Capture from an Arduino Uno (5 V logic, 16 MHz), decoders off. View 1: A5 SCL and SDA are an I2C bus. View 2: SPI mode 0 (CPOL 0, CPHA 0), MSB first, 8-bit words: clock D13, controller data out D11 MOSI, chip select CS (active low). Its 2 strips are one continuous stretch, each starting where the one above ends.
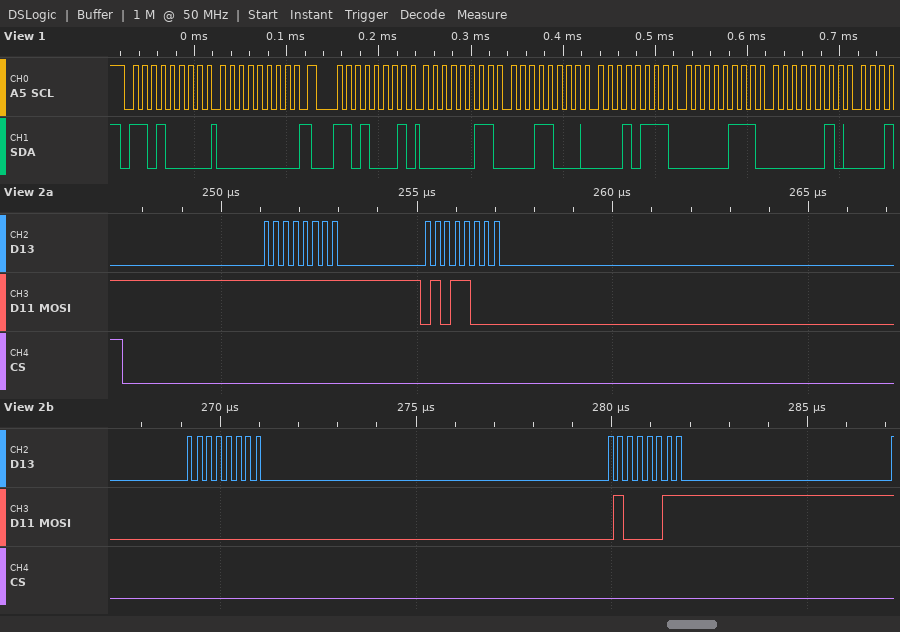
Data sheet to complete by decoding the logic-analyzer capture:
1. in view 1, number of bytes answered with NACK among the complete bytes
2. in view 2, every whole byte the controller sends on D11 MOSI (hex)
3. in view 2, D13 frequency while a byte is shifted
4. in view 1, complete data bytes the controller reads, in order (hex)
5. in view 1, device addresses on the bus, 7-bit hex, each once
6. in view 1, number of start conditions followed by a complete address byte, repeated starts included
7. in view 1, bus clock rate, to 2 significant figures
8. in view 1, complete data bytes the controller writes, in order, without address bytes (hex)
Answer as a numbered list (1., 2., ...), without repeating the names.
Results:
1. 0
2. 0xFF 0x58 0x00 0x43
3. 4 MHz
4. 03 18 17 07 02
5. 0x68
6. 2
7. 100 kHz
8. 00
